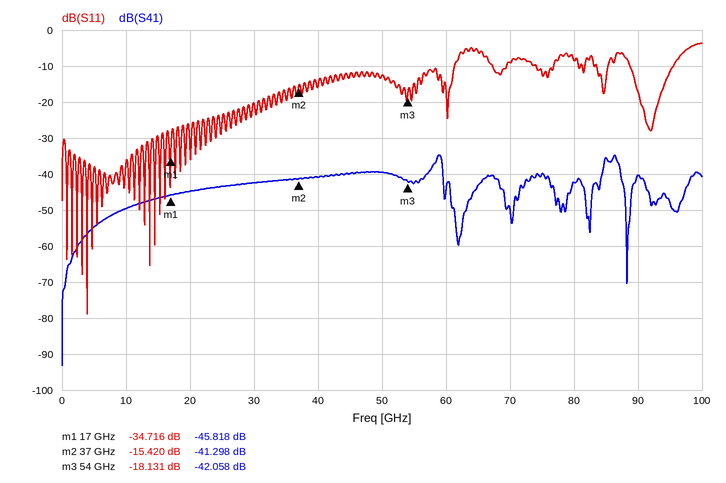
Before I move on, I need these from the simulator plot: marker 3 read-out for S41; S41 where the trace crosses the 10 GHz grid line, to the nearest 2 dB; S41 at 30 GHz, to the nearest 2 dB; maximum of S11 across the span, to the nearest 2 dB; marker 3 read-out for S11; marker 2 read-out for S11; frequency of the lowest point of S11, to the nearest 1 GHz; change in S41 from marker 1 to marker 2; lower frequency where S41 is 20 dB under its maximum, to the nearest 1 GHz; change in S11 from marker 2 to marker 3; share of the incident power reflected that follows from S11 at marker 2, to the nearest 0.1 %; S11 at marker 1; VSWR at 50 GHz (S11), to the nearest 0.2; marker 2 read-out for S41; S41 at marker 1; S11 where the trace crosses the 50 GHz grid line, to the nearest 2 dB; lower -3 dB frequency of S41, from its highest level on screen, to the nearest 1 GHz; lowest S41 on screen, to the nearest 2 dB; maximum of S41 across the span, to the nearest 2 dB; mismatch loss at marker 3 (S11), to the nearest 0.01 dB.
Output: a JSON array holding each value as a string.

["-42.058 dB", "-50 dB", "-42 dB", "-4 dB", "-18.131 dB", "-15.420 dB", "4 GHz", "4.520 dB", "5 GHz", "-2.711 dB", "2.9 %", "-34.716 dB", "1.6", "-41.298 dB", "-45.818 dB", "-12 dB", "58 GHz", "-94 dB", "-34 dB", "0.07 dB"]
